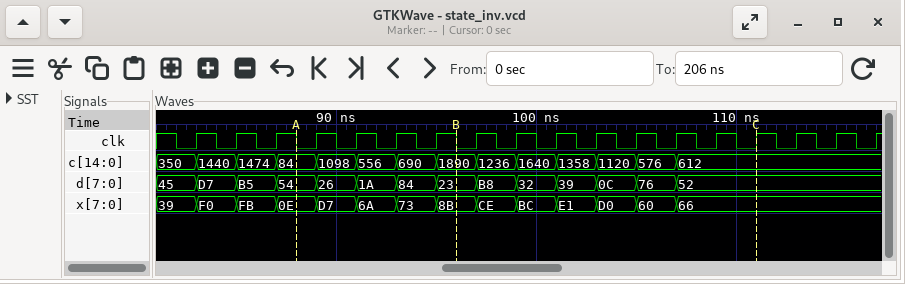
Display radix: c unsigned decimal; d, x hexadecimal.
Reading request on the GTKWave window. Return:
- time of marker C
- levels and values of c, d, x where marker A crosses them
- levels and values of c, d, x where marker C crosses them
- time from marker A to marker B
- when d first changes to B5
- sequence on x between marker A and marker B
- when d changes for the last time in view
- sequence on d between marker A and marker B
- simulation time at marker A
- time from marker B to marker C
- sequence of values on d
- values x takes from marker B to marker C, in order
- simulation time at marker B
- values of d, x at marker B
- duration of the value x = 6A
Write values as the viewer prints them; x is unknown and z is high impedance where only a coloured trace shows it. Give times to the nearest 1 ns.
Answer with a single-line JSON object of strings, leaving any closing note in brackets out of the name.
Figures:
{"time of marker C": "111 ns", "levels and values of c, d, x where marker A crosses them": "c=84, d=54, x=0E", "levels and values of c, d, x where marker C crosses them": "c=612, d=52, x=66", "time from marker A to marker B": "8 ns", "when d first changes to B5": "85 ns", "sequence on x between marker A and marker B": "0E, D7, 6A, 73, 8B", "when d changes for the last time in view": "107 ns", "sequence on d between marker A and marker B": "54, 26, 1A, 84, 23", "simulation time at marker A": "88 ns", "time from marker B to marker C": "15 ns", "sequence of values on d": "45, D7, B5, 54, 26, 1A, 84, 23, B8, 32, 39, 0C, 76, 52", "values x takes from marker B to marker C, in order": "8B, CE, BC, E1, D0, 60, 66", "simulation time at marker B": "96 ns", "values of d, x at marker B": "d=23, x=8B", "duration of the value x = 6A": "2 ns"}
